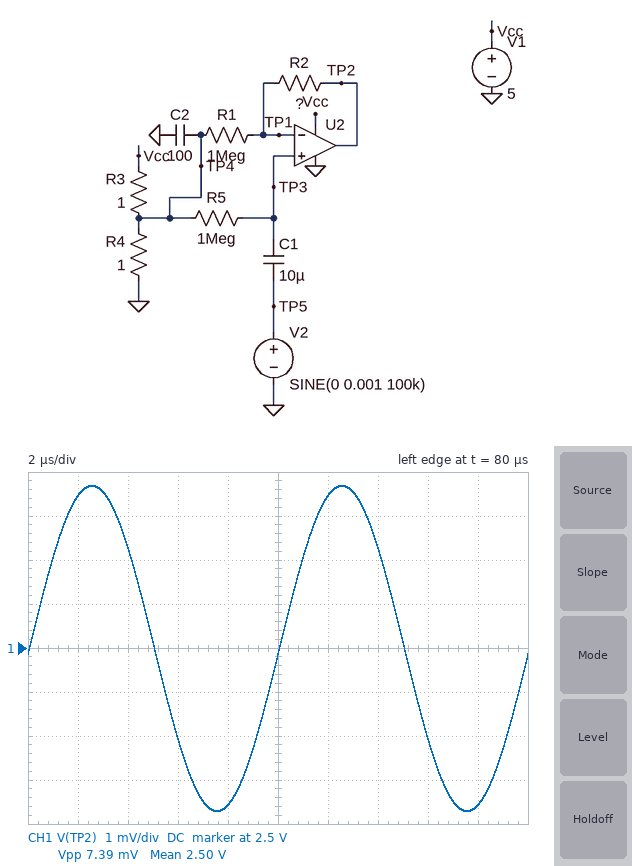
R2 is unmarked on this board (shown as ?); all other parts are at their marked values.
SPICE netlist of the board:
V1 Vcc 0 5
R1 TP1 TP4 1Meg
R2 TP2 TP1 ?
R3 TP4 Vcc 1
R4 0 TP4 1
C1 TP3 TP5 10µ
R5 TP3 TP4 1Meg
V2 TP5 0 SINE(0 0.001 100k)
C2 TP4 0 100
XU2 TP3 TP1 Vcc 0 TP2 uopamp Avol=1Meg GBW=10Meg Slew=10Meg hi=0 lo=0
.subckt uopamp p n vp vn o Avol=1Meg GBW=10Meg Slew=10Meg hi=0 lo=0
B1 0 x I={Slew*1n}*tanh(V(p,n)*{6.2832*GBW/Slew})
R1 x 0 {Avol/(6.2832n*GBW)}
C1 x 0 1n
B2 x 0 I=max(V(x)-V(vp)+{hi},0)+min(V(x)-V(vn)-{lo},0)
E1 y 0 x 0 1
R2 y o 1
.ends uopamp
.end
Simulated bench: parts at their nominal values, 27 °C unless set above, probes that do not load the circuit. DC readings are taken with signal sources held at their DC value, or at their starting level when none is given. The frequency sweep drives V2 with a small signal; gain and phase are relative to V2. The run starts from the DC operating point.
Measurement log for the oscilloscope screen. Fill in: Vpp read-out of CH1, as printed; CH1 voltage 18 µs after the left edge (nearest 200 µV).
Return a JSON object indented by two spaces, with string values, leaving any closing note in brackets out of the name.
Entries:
{
  "Vpp read-out of CH1, as printed": "7.39 mV",
  "CH1 voltage 18 µs after the left edge": "2.4964 V"
}
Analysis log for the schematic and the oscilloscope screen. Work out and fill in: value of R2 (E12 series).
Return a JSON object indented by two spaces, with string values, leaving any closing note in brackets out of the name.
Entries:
{
  "value of R2": "2.7 MΩ"
}
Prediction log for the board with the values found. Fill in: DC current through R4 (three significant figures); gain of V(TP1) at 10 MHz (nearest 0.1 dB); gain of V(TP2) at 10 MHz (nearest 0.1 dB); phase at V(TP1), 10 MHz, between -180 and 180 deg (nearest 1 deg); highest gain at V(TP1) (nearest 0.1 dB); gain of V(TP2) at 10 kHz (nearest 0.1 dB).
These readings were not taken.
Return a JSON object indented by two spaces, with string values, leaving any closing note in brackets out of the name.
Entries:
{
  "DC current through R4": "2.50 A",
  "gain of V(TP1) at 10 MHz": "-11.7 dB",
  "gain of V(TP2) at 10 MHz": "-0.3 dB",
  "phase at V(TP1), 10 MHz, between -180 and 180 deg": "-75 deg",
  "highest gain at V(TP1)": "0 dB",
  "gain of V(TP2) at 10 kHz": "11.4 dB"
}
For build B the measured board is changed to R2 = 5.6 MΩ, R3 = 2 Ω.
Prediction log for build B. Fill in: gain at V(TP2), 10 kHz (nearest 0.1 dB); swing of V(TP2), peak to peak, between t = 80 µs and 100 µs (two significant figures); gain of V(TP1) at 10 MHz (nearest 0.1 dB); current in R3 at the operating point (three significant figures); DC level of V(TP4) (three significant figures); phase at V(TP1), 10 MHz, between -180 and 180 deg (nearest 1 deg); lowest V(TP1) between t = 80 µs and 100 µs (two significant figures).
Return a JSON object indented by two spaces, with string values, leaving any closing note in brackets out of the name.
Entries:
{
  "gain at V(TP2), 10 kHz": "16.4 dB",
  "swing of V(TP2), peak to peak, between t = 80 µs and 100 µs": "13 mV",
  "gain of V(TP1) at 10 MHz": "-16.5 dB",
  "current in R3 at the operating point": "1.67 A",
  "DC level of V(TP4)": "1.67 V",
  "phase at V(TP1), 10 MHz, between -180 and 180 deg": "-81 deg",
  "lowest V(TP1) between t = 80 µs and 100 µs": "1.7 V"
}
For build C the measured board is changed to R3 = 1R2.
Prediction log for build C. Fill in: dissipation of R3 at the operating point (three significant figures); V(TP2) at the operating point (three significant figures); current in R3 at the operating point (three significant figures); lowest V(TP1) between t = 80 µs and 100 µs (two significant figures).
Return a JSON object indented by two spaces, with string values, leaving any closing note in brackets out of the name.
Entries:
{
  "dissipation of R3 at the operating point": "6.20 W",
  "V(TP2) at the operating point": "2.27 V",
  "current in R3 at the operating point": "2.27 A",
  "lowest V(TP1) between t = 80 µs and 100 µs": "2.3 V"
}
